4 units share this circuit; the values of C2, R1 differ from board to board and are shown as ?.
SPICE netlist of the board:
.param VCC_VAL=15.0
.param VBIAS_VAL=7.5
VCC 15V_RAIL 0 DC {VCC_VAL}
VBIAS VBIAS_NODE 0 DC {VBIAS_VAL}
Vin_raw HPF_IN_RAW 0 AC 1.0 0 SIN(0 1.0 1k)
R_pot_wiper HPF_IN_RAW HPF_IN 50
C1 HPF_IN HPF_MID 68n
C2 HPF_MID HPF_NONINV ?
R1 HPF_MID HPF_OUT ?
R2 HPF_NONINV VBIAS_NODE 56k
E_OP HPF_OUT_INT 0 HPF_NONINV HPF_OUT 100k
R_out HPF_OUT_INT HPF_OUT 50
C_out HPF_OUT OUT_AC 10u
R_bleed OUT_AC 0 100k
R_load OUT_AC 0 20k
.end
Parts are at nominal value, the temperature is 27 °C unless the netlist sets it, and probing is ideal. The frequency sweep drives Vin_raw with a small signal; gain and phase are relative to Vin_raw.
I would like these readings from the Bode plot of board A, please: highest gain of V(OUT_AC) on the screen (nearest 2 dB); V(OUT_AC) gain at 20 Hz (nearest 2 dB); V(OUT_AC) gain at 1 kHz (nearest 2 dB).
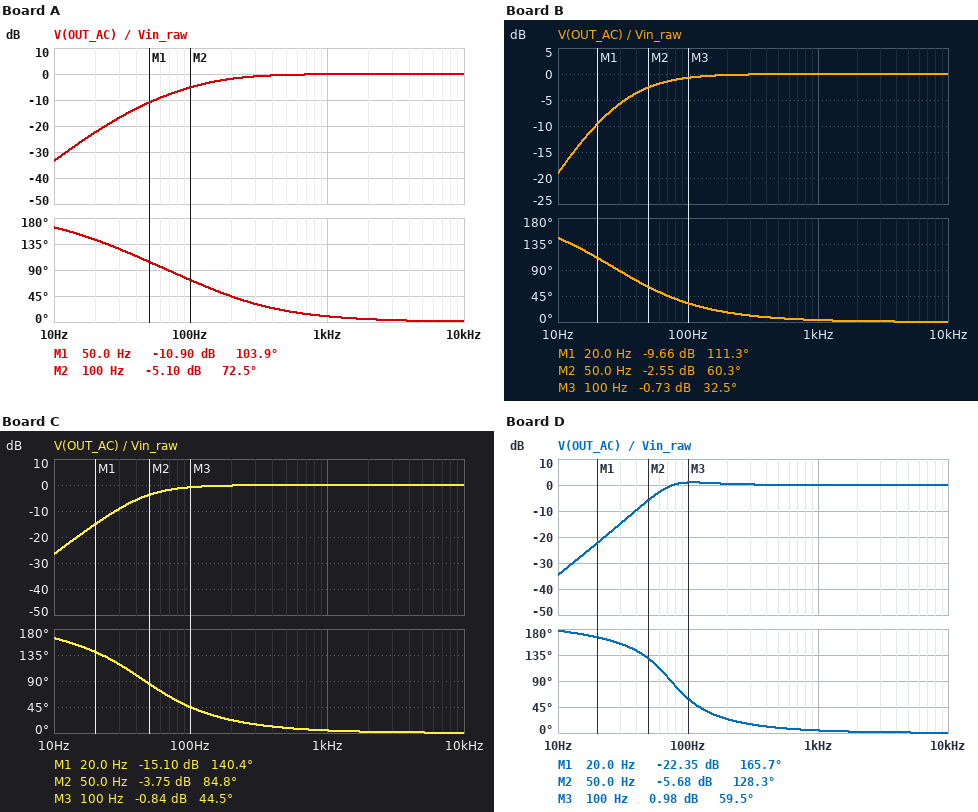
0 dB
-22 dB
0 dB
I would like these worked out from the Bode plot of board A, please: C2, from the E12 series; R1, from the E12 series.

22 nF
68 kΩ
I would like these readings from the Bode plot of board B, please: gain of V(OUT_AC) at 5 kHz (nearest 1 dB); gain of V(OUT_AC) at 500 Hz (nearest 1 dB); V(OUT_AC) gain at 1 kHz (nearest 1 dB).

0 dB
0 dB
0 dB
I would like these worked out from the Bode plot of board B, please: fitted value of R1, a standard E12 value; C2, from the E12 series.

47 kΩ
180 nF
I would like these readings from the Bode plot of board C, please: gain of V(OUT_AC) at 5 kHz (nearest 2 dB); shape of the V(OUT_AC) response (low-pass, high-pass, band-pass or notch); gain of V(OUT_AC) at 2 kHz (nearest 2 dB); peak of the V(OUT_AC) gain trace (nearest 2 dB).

0 dB
high-pass
0 dB
0 dB
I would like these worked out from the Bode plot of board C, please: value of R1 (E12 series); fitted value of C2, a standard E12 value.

39 kΩ
82 nF
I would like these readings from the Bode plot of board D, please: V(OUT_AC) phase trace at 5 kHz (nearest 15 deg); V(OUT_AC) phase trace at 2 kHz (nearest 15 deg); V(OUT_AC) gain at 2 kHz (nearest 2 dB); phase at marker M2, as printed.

0 deg
0 deg
0 dB
128.3 deg
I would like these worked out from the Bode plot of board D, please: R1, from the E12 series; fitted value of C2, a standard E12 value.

15 kΩ
82 nF
